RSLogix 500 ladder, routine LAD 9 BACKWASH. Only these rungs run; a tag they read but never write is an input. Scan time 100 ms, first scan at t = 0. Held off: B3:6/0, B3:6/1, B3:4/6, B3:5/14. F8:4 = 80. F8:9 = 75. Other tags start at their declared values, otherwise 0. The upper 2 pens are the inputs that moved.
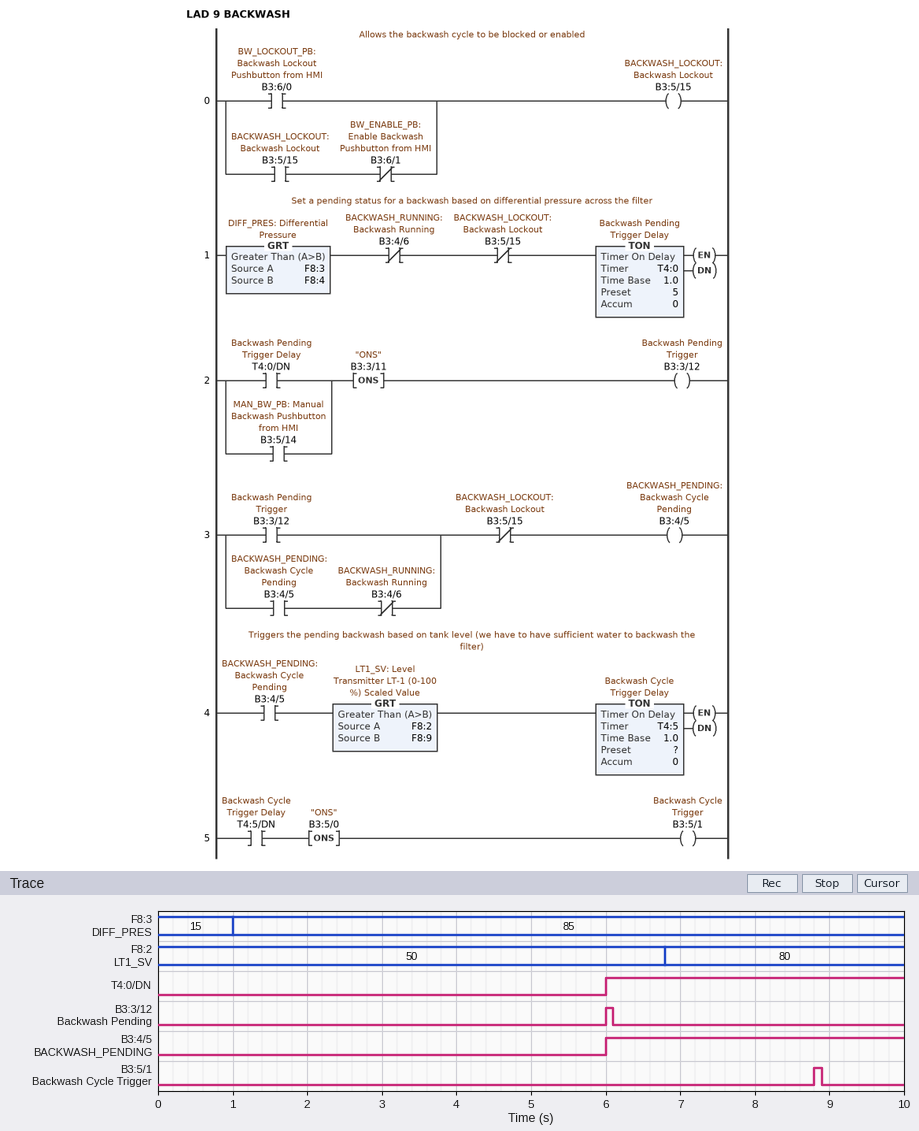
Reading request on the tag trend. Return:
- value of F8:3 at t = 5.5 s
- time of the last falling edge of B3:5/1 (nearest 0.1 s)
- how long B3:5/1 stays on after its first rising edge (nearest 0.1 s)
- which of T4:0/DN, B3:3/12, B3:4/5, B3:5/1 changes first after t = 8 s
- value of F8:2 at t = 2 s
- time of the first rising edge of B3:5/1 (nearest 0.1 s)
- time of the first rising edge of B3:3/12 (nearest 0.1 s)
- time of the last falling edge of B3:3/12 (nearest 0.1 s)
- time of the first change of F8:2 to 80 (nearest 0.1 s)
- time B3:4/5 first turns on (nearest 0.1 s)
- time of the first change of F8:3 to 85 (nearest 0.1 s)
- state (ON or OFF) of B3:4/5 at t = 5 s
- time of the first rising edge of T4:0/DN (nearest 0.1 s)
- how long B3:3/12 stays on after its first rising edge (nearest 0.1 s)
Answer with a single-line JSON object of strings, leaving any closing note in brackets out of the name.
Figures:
{"value of F8:3 at t = 5.5 s": "85", "time of the last falling edge of B3:5/1": "8.9 s", "how long B3:5/1 stays on after its first rising edge": "0.1 s", "which of T4:0/DN, B3:3/12, B3:4/5, B3:5/1 changes first after t = 8 s": "B3:5/1", "value of F8:2 at t = 2 s": "50", "time of the first rising edge of B3:5/1": "8.8 s", "time of the first rising edge of B3:3/12": "6.0 s", "time of the last falling edge of B3:3/12": "6.1 s", "time of the first change of F8:2 to 80": "6.8 s", "time B3:4/5 first turns on": "6.0 s", "time of the first change of F8:3 to 85": "1.0 s", "state (ON or OFF) of B3:4/5 at t = 5 s": "OFF", "time of the first rising edge of T4:0/DN": "6.0 s", "how long B3:3/12 stays on after its first rising edge": "0.1 s"}
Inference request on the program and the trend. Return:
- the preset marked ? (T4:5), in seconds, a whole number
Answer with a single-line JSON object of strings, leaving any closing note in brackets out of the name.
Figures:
{"the preset marked ? (T4:5), in seconds, a whole number": "2 s"}
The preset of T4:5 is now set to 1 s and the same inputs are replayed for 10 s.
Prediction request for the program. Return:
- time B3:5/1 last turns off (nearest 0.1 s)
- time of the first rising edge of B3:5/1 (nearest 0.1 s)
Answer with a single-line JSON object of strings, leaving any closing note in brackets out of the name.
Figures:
{"time B3:5/1 last turns off": "7.9 s", "time of the first rising edge of B3:5/1": "7.8 s"}
